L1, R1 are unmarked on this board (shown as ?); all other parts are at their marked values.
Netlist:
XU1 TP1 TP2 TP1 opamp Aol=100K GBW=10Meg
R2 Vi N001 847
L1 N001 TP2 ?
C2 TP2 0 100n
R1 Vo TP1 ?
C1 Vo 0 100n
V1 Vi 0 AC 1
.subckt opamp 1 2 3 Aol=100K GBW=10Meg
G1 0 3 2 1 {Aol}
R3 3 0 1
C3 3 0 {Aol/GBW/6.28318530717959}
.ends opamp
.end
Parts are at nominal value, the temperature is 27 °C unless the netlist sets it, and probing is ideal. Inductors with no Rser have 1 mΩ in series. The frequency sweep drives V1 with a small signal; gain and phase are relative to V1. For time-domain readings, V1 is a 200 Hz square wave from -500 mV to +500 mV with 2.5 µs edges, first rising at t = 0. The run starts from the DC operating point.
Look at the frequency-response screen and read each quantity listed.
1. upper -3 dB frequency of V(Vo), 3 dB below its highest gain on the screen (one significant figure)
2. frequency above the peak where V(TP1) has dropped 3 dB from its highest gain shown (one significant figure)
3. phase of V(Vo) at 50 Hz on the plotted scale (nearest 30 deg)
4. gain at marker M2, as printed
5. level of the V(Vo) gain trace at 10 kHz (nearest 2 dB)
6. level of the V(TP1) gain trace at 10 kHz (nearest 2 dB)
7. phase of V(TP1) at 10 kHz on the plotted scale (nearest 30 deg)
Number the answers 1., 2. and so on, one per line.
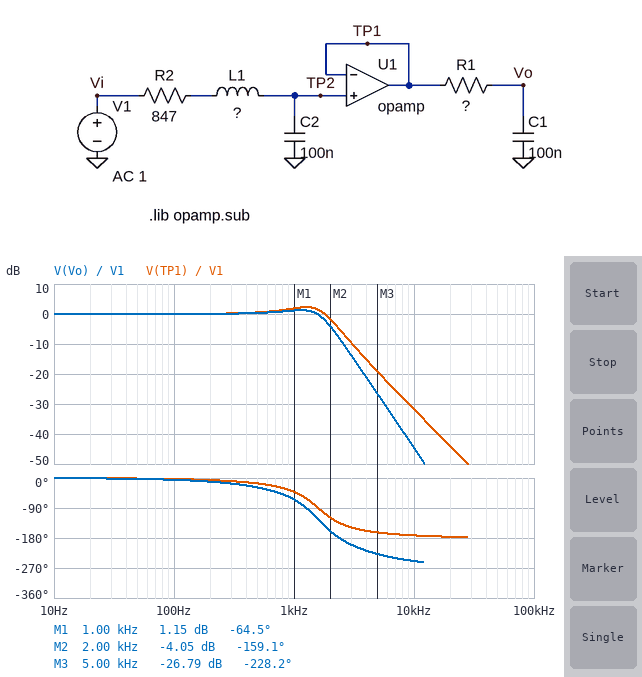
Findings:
1. 2 kHz
2. 2 kHz
3. 0 deg
4. -4.05 dB
5. -44 dB
6. -32 dB
7. -180 deg
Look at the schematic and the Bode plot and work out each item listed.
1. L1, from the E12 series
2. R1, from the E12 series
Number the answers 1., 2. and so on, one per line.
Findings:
1. 100 mH
2. 680 Ω
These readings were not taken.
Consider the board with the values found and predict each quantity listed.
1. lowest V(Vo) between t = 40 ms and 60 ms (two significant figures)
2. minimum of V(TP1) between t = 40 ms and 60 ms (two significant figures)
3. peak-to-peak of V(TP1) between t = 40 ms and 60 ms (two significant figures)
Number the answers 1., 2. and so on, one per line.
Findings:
1. -680 mV
2. -730 mV
3. 1.5 V
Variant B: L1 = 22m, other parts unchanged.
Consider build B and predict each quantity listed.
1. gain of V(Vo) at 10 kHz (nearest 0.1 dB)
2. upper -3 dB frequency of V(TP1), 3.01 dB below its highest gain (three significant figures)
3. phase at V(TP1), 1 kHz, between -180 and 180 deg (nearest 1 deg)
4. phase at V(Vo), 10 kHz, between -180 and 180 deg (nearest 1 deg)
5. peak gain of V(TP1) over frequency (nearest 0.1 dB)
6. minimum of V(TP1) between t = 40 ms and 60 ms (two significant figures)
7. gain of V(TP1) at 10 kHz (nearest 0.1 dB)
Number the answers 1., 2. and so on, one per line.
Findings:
1. -32.3 dB
2. 2.52 kHz
3. -30 deg
4. 138 deg
5. 0 dB
6. -500 mV
7. -19.4 dB
